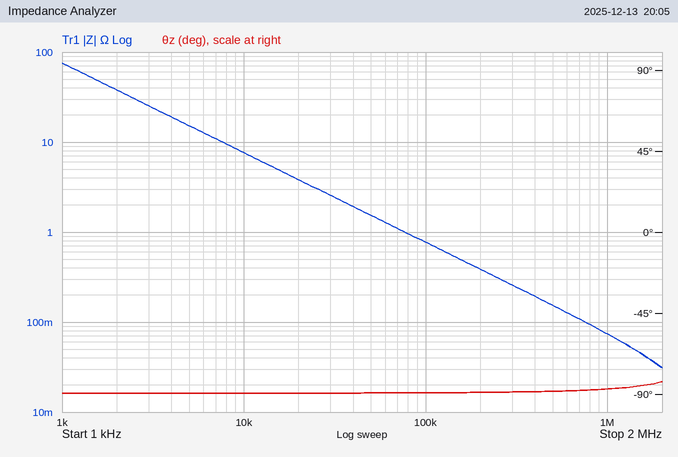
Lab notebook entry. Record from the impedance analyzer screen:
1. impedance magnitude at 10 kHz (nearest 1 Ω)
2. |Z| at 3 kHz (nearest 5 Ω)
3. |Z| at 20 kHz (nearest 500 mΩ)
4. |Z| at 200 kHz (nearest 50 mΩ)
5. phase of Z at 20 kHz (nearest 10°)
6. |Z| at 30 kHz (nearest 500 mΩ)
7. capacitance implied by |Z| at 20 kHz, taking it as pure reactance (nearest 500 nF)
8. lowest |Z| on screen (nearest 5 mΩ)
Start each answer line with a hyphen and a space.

- 8 Ω
- 25 Ω
- 4.0 Ω
- 400 mΩ
- -90°
- 2.5 Ω
- 2.0 µF
- 30 mΩ
